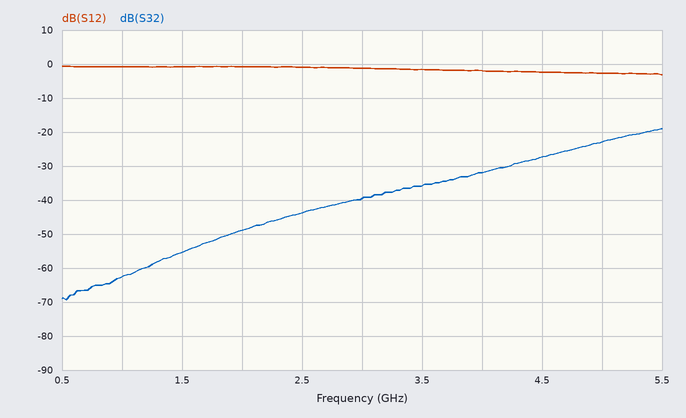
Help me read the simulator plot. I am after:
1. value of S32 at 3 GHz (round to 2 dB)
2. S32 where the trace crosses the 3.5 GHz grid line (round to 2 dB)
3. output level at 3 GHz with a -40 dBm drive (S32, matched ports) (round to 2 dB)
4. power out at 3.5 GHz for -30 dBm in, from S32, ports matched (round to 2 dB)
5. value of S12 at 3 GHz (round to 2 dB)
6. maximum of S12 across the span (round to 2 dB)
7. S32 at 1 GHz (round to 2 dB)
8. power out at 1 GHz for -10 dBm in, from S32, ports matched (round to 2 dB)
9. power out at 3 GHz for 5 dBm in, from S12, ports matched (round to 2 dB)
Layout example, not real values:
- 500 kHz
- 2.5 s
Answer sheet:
- -40 dB
- -36 dB
- -80 dBm
- -66 dBm
- -2 dB
- 0 dB
- -62 dB
- -72 dBm
- 4 dBm
